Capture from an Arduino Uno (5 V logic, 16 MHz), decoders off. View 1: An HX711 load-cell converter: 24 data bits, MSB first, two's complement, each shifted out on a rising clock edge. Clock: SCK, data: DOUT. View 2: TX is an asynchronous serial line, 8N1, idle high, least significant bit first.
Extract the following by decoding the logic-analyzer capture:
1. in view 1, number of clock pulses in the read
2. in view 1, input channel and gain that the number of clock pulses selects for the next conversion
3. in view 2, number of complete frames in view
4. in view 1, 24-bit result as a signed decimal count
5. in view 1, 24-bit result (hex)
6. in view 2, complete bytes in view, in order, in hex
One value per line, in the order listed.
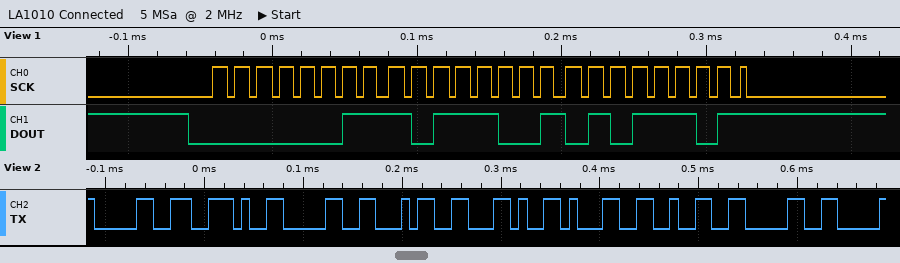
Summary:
25
channel A, gain 128
8
244061
0x03B95D
30 2E 30 34 2C 31 32 30
